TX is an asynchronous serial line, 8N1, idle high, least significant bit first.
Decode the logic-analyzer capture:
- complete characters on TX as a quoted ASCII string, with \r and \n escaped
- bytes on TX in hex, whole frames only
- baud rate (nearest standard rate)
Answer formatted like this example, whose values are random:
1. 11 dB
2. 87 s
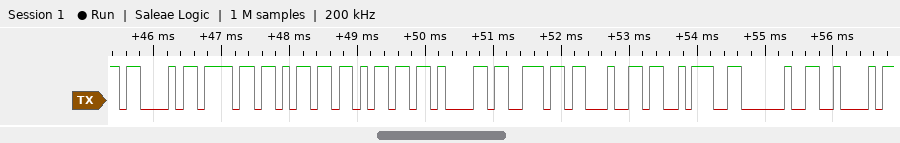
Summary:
1. "Command: B"
2. 0x43 0x6F 0x6D 0x6D 0x61 0x6E 0x64 0x3A 0x20 0x42
3. 9600 baud
